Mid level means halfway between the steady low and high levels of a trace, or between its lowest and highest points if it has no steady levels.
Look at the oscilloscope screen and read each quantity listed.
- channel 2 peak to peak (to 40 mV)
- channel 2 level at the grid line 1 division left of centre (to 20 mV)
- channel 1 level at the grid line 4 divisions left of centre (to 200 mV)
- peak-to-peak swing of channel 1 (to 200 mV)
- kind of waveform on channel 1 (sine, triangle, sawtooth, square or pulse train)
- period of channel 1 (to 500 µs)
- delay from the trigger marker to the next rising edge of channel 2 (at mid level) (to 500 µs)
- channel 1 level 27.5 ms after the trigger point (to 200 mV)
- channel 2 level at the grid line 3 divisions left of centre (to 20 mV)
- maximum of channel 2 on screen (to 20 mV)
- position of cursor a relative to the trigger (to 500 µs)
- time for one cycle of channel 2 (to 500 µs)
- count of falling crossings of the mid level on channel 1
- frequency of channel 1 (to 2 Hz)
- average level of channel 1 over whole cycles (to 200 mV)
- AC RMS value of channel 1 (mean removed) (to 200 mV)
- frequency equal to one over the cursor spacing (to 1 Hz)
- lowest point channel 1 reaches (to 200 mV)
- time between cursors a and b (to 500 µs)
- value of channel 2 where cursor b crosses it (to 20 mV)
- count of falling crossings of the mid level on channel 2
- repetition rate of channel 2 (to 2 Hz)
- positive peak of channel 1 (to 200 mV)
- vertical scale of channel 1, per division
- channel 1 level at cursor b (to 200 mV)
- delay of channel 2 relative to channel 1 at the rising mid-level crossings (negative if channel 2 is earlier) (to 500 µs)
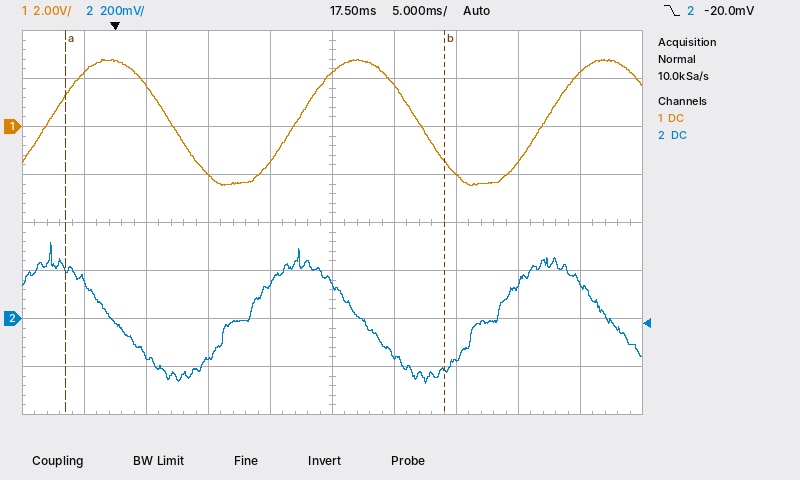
600 mV
140 mV
2.2 V
5.2 V
sine
20.0 ms
11.0 ms
-2.0 V
-160 mV
320 mV
-4.0 ms
20.0 ms
2
50 Hz
200 mV
1.8 V
33 Hz
-2.4 V
30.5 ms
-220 mV
3
50 Hz
2.8 V
2 V
-1.4 V
-3.5 ms
